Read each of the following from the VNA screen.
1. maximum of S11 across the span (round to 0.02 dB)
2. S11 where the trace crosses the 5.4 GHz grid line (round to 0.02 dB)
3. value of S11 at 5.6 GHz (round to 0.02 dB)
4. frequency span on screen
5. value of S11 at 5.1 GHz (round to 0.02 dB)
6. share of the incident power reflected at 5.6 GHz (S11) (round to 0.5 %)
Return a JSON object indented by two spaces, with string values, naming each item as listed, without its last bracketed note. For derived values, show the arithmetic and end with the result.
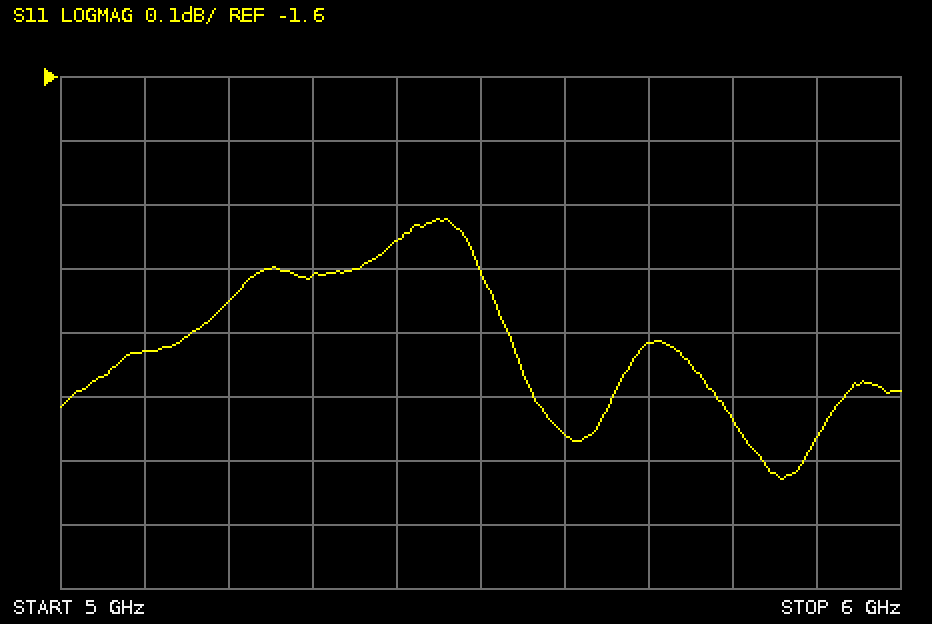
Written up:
{
  "maximum of S11 across the span": "-1.82 dB",
  "S11 where the trace crosses the 5.4 GHz grid line": "-1.86 dB",
  "value of S11 at 5.6 GHz": "-2.16 dB",
  "frequency span on screen": "1 GHz",
  "value of S11 at 5.1 GHz": "-2.02 dB",
  "share of the incident power reflected at 5.6 GHz (S11)": "10^(-2.16/10) ≈ 60.8 %, so 61.0 % to the nearest 0.5 %"
}
